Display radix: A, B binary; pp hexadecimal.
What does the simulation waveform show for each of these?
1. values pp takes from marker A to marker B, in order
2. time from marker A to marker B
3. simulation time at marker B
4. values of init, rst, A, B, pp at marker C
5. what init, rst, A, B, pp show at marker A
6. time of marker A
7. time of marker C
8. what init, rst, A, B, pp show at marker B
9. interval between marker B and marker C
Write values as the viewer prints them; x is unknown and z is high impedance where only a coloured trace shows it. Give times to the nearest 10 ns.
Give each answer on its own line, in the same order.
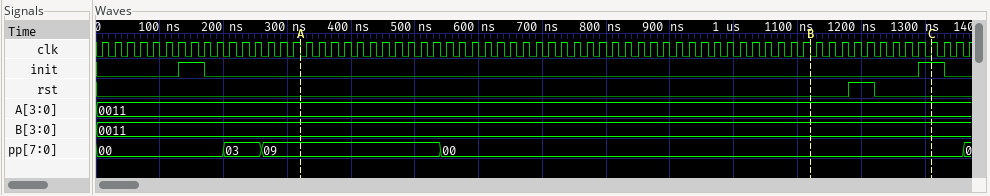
09, 00
800 ns
1120 ns
init=1, rst=0, A=0011, B=0011, pp=00
init=0, rst=0, A=0011, B=0011, pp=09
320 ns
1310 ns
init=0, rst=0, A=0011, B=0011, pp=00
190 ns
